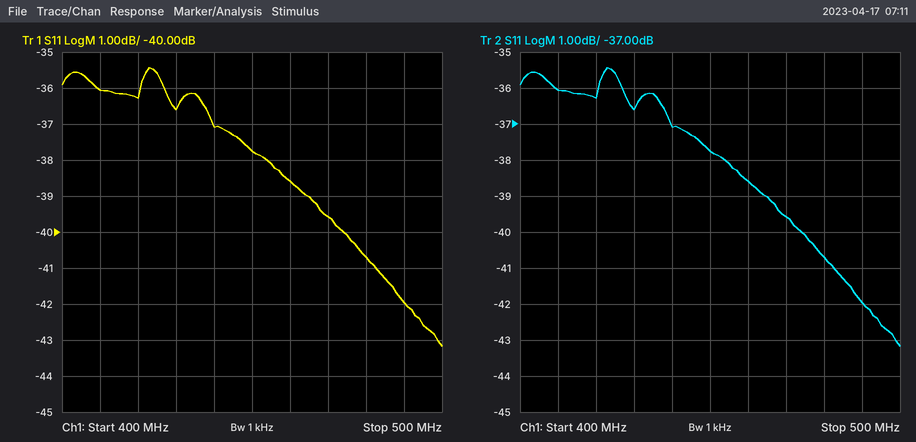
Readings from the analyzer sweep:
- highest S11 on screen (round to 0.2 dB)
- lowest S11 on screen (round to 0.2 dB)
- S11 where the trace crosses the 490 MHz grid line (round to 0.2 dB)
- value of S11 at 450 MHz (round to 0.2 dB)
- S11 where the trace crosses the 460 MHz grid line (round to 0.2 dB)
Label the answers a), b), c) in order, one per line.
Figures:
a) -35.4 dB
b) -43.2 dB
c) -42.0 dB
d) -37.8 dB
e) -38.6 dB
